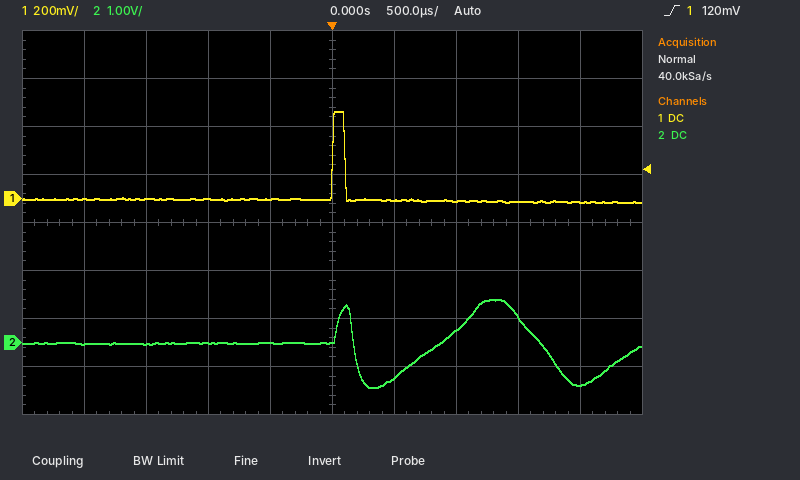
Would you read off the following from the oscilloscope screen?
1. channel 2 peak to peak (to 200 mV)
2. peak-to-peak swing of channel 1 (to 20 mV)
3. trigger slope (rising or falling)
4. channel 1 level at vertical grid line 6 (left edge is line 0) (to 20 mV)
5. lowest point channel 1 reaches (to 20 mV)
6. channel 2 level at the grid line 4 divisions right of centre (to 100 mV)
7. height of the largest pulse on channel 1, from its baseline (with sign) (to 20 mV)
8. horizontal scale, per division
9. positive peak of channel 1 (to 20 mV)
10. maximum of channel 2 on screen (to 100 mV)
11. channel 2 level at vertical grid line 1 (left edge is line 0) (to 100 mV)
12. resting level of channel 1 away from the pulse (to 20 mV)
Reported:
1.8 V
380 mV
rising
0 mV
-20 mV
-900 mV
+360 mV
500 µs
360 mV
900 mV
0.0 V
0 mV
